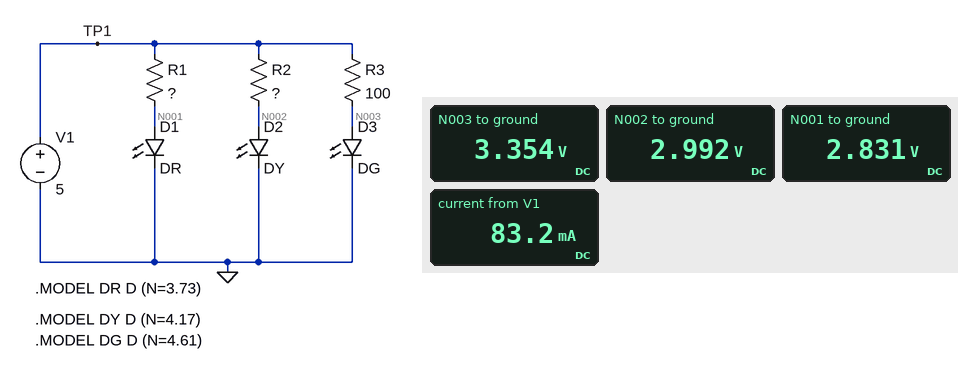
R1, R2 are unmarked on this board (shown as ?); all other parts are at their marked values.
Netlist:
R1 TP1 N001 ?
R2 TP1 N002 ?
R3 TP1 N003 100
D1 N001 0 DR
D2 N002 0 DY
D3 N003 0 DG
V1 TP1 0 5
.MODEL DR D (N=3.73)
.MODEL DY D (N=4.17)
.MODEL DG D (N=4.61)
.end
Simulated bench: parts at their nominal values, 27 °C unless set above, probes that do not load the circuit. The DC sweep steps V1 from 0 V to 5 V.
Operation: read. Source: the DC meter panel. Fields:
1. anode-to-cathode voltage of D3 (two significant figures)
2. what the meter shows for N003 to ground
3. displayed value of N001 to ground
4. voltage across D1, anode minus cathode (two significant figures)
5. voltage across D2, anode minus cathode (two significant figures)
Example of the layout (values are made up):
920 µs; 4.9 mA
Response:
3.4 V; 3.354 V; 2.831 V; 2.8 V; 3.0 V
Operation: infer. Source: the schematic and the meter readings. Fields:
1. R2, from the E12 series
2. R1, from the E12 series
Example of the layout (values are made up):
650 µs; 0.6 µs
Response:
180 Ω; 39 Ω
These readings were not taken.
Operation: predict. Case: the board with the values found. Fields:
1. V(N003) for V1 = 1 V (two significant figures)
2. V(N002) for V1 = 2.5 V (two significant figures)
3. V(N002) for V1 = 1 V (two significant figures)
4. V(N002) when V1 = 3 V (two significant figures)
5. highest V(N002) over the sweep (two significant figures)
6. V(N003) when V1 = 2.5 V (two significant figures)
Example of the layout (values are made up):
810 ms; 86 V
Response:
1.0 V; 2.5 V; 1.0 V; 2.8 V; 3.0 V; 2.5 V
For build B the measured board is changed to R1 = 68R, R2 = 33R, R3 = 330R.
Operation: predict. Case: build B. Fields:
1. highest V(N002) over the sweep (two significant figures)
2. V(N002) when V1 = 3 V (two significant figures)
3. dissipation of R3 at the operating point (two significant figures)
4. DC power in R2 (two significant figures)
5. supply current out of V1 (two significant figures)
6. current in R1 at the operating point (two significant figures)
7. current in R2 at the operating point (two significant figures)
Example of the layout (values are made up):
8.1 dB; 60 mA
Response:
3.2 V; 2.9 V; 9.6 mW; 100 mW; 94 mA; 33 mA; 56 mA
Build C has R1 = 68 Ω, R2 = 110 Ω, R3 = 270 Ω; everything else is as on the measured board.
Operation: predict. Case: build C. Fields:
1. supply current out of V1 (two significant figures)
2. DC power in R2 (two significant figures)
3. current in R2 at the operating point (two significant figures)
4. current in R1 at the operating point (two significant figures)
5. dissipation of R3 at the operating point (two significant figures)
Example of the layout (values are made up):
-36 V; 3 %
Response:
57 mA; 35 mW; 18 mA; 33 mA; 11 mW
